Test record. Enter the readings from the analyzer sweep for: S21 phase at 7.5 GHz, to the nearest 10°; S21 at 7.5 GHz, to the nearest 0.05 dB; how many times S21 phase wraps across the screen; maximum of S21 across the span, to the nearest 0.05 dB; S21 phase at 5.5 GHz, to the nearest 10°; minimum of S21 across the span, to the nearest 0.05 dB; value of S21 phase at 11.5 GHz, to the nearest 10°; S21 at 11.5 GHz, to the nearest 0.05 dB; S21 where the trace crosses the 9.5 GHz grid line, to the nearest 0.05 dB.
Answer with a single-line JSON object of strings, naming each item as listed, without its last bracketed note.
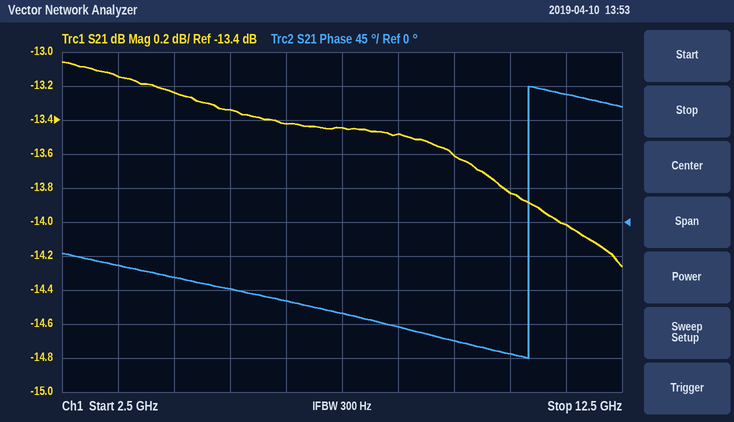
{"S21 phase at 7.5 GHz, to the nearest 10°": "-120°", "S21 at 7.5 GHz, to the nearest 0.05 dB": "-13.45 dB", "how many times S21 phase wraps across the screen": "1", "maximum of S21 across the span, to the nearest 0.05 dB": "-13.05 dB", "S21 phase at 5.5 GHz, to the nearest 10°": "-90°", "minimum of S21 across the span, to the nearest 0.05 dB": "-14.25 dB", "value of S21 phase at 11.5 GHz, to the nearest 10°": "170°", "S21 at 11.5 GHz, to the nearest 0.05 dB": "-14.00 dB", "S21 where the trace crosses the 9.5 GHz grid line, to the nearest 0.05 dB": "-13.60 dB"}
